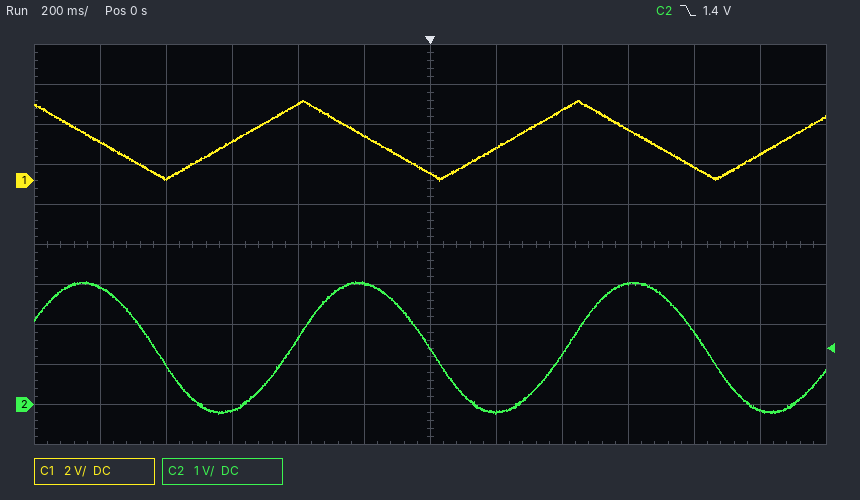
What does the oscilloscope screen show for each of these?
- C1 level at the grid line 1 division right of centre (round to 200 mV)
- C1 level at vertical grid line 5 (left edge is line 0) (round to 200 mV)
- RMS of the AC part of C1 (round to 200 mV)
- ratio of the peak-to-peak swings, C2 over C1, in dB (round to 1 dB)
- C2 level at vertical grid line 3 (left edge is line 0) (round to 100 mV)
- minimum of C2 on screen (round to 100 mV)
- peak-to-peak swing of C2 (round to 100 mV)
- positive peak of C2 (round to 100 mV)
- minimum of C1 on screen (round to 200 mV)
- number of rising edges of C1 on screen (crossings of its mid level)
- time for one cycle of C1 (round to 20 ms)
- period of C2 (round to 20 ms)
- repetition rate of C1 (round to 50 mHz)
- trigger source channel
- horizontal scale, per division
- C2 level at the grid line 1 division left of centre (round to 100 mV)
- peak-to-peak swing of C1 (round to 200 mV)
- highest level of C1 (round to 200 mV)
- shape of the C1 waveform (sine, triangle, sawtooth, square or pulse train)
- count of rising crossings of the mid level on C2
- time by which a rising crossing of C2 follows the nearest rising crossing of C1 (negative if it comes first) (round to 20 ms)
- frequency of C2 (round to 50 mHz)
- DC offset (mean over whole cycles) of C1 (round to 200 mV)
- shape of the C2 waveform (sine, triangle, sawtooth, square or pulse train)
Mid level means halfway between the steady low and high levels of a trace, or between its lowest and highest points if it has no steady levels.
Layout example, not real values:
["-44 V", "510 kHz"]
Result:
["1.6 V", "2.2 V", "1.2 V", "-2 dB", "-200 mV", "-200 mV", "3.3 V", "3.1 V", "0.0 V", "3", "840 ms", "840 ms", "1.20 Hz", "C2", "200 ms", "3.0 V", "4.0 V", "4.0 V", "triangle", "2", "+180 ms", "1.20 Hz", "2.0 V", "sine"]
